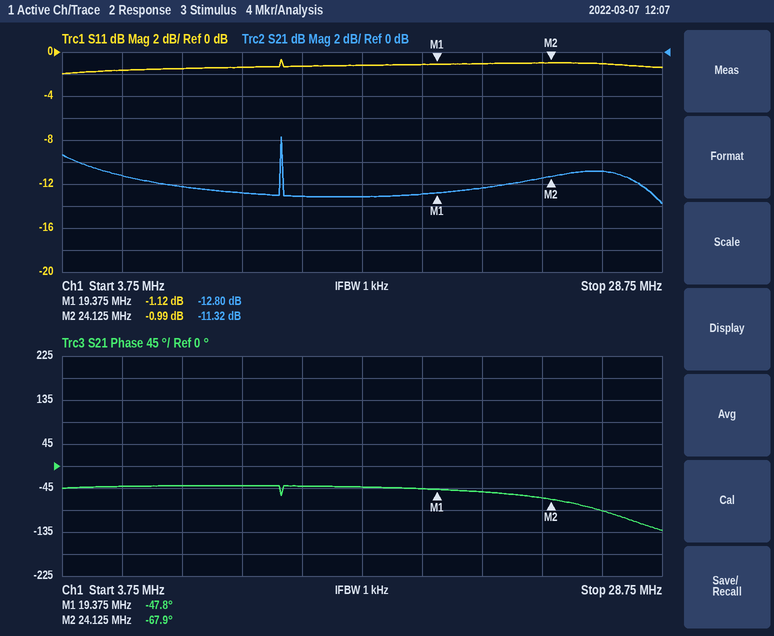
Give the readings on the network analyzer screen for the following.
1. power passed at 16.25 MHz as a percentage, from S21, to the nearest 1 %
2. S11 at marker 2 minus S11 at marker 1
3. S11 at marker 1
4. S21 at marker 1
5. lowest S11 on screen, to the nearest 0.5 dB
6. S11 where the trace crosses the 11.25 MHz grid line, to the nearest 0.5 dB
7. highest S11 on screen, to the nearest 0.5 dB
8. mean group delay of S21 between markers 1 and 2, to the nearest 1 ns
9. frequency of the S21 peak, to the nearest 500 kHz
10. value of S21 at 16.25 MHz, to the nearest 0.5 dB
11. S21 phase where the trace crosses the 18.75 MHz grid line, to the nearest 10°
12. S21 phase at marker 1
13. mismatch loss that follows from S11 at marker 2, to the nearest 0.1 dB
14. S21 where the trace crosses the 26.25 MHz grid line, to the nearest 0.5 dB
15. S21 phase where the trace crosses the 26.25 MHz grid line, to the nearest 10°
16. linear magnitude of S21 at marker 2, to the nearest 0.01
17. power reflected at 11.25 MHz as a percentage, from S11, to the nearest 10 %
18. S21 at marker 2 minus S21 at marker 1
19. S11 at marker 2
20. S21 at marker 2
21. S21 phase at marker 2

5 %
0.13 dB
-1.12 dB
-12.80 dB
-2.0 dB
-1.5 dB
-0.5 dB
12 ns
13.0 MHz
-13.0 dB
-50°
-47.8°
6.9 dB
-11.0 dB
-90°
0.27
70 %
1.48 dB
-0.99 dB
-11.32 dB
-67.9°
